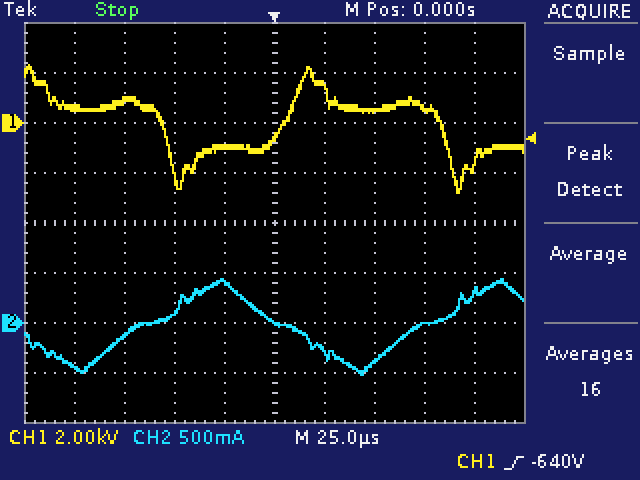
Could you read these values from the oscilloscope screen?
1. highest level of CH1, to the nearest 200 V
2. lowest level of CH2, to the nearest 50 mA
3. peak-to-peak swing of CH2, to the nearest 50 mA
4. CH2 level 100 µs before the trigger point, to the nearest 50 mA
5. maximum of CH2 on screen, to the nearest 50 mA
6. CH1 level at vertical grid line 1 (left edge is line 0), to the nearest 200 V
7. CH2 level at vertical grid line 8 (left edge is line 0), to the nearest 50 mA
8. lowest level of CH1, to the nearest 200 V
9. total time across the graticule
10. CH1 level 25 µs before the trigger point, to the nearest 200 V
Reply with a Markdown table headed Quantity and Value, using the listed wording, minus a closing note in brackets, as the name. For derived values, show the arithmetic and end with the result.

| Quantity | Value |
|---|---|
| highest level of CH1, to the nearest 200 V | 2.4 kV |
| lowest level of CH2, to the nearest 50 mA | -500 mA |
| peak-to-peak swing of CH2, to the nearest 50 mA | 450 mA − (-500 mA) = 950 mA |
| CH2 level 100 µs before the trigger point, to the nearest 50 mA | -450 mA |
| maximum of CH2 on screen, to the nearest 50 mA | 450 mA |
| CH1 level at vertical grid line 1 (left edge is line 0), to the nearest 200 V | 600 V |
| CH2 level at vertical grid line 8 (left edge is line 0), to the nearest 50 mA | 0 mA |
| lowest level of CH1, to the nearest 200 V | -2.8 kV |
| total time across the graticule | 250 µs |
| CH1 level 25 µs before the trigger point, to the nearest 200 V | -1.0 kV |
